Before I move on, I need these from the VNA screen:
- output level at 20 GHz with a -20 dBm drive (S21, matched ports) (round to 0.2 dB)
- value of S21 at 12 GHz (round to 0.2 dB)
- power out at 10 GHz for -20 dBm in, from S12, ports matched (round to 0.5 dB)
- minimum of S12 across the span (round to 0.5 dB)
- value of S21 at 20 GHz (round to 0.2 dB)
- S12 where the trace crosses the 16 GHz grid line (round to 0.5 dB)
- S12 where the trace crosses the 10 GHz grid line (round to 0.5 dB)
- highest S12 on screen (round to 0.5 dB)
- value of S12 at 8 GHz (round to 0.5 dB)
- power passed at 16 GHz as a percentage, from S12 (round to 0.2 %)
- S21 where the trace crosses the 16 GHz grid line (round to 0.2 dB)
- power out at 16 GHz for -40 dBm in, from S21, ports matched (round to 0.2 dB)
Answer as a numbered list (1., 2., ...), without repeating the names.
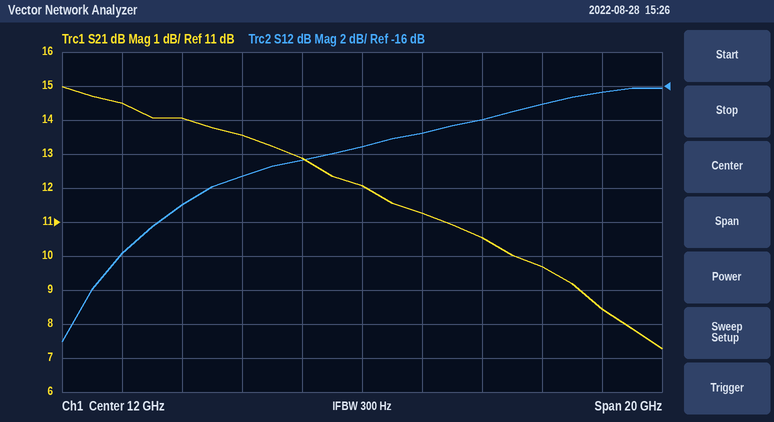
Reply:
1. -11.6 dBm
2. 12.0 dB
3. -40.5 dBm
4. -31.0 dB
5. 8.4 dB
6. -18.0 dB
7. -20.5 dB
8. -16.0 dB
9. -21.5 dB
10. 1.6 %
11. 10.6 dB
12. -29.4 dBm
